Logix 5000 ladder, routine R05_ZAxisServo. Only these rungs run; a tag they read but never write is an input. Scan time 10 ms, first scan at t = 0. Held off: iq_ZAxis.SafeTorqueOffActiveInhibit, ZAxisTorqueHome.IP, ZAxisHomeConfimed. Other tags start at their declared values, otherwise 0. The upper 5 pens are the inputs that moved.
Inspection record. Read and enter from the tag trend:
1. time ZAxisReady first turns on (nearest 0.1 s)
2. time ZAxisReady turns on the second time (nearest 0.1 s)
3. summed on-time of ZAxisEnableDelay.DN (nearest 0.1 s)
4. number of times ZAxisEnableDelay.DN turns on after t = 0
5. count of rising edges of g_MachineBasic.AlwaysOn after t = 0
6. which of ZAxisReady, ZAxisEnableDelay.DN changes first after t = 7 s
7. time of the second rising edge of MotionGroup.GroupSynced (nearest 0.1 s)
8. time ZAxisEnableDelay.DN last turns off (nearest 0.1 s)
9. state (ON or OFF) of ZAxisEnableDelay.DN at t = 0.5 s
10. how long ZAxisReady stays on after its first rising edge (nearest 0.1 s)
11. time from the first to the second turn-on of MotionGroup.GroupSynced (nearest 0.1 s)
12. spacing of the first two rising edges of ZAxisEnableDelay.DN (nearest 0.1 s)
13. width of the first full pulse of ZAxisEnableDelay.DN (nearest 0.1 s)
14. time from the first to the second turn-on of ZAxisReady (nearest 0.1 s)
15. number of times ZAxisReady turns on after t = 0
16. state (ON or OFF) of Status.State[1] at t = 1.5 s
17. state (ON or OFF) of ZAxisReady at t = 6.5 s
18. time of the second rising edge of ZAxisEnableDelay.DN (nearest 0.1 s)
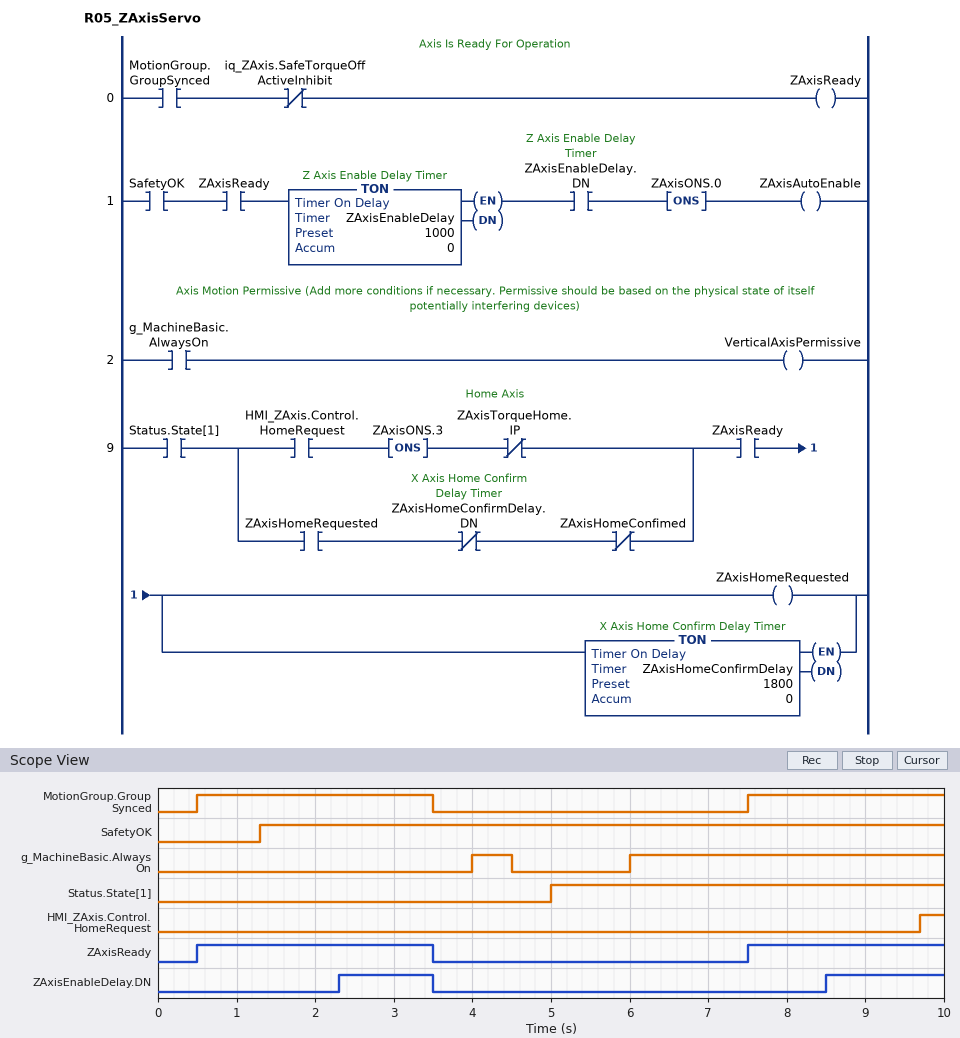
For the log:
0.5 s
7.5 s
2.7 s
2
2
ZAxisReady
7.5 s
3.5 s
OFF
3.0 s
7.0 s
6.2 s
1.2 s
7.0 s
2
OFF
OFF
8.5 s
